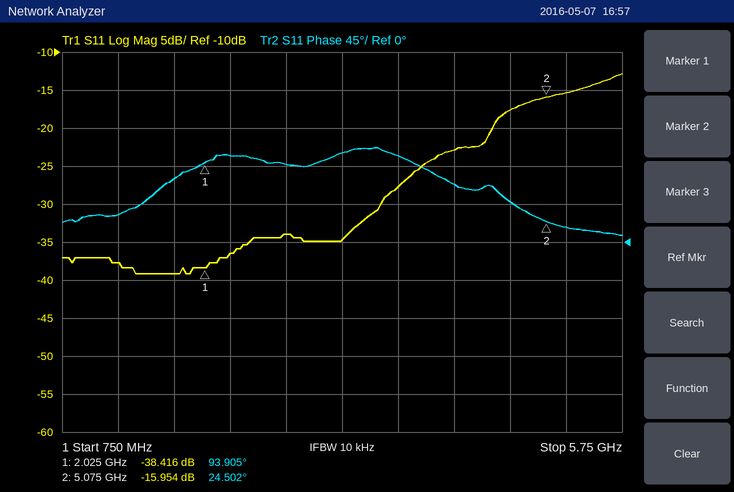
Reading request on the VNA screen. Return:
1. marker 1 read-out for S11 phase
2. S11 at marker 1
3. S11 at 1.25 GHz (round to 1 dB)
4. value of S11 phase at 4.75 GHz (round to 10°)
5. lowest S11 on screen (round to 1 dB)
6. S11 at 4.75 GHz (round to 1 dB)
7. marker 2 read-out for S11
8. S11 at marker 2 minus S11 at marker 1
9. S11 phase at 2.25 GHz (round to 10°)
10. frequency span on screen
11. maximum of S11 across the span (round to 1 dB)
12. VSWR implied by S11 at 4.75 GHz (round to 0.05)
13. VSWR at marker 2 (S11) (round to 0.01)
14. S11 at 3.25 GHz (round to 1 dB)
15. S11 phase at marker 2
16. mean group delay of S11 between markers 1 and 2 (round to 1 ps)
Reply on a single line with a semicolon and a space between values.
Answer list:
93.905°; -38.416 dB; -38 dB; 50°; -39 dB; -18 dB; -15.954 dB; 22.462 dB; 100°; 5 GHz; -13 dB; 1.30; 1.38; -35 dB; 24.502°; 63 ps
